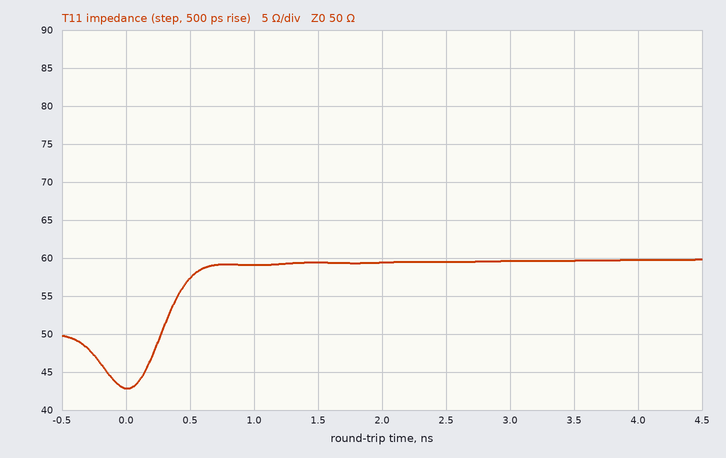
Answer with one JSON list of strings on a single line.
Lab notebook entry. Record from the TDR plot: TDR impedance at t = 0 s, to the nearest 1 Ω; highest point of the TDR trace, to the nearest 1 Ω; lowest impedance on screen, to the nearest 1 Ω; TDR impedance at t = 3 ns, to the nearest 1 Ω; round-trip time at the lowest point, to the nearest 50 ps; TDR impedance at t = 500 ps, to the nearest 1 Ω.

["43 Ω", "60 Ω", "43 Ω", "60 Ω", "0 ps", "57 Ω"]
